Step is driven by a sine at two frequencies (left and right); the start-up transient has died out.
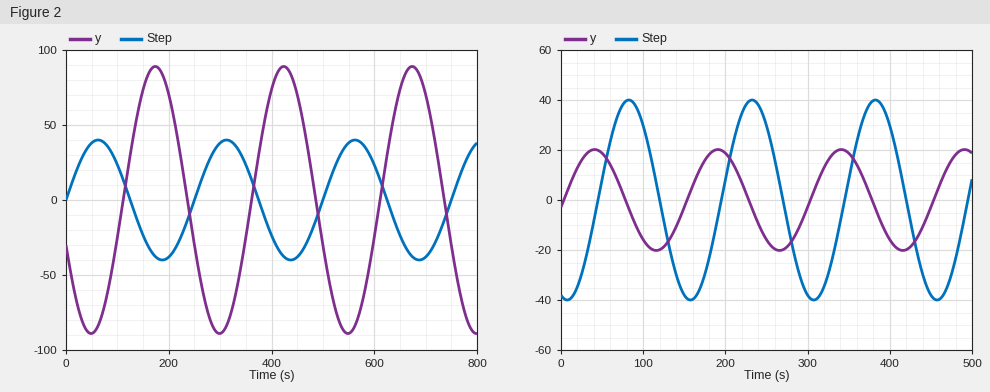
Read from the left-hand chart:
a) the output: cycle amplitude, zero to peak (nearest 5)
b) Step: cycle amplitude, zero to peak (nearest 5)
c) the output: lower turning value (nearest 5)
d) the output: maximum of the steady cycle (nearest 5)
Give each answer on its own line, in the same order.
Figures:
90
40
-90
90
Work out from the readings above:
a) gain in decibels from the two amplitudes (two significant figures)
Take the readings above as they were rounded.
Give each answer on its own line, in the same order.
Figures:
7.0 dB
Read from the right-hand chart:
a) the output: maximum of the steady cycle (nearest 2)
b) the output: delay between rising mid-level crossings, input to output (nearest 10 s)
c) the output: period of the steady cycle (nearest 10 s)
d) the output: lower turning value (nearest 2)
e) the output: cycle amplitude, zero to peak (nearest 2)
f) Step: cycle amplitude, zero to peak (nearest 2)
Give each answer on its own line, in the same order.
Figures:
20
110 s
150 s
-20
20
40
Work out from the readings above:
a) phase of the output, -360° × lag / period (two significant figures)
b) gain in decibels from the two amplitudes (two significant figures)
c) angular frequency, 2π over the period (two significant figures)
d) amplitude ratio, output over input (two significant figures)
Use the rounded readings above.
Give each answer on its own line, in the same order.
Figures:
-260°
-6.0 dB
0.042 rad/s
0.50
